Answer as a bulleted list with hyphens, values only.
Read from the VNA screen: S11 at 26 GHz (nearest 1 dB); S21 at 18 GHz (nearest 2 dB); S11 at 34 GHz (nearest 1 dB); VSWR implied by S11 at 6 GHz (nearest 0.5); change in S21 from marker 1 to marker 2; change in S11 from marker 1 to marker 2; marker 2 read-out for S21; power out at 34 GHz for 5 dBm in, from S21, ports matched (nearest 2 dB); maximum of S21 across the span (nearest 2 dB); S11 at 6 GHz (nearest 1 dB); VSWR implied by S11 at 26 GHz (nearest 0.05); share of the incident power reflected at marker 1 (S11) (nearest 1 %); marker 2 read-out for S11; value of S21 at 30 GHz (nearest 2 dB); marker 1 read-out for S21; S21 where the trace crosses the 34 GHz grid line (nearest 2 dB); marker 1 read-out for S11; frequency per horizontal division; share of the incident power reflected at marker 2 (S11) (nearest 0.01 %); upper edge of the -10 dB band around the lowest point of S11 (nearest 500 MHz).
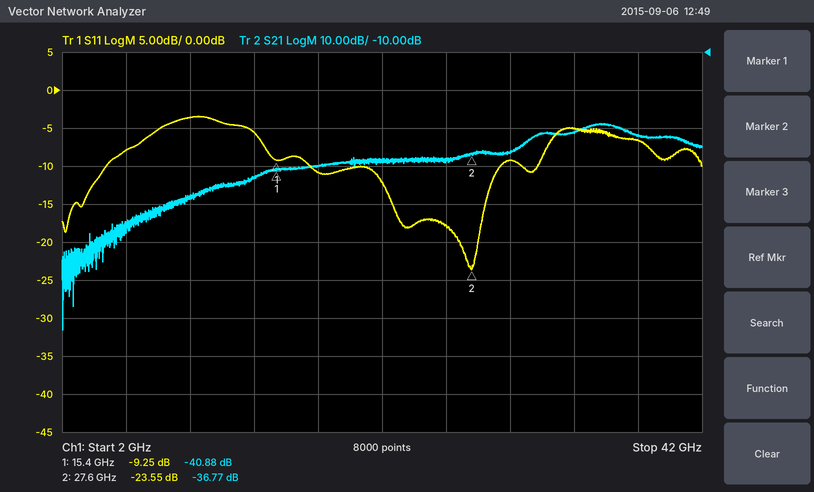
- -18 dB
- -40 dB
- -5 dB
- 2.5
- 4.11 dB
- -14.30 dB
- -36.77 dB
- -26 dBm
- -28 dB
- -8 dB
- 1.30
- 12 %
- -23.55 dB
- -36 dB
- -40.88 dB
- -32 dB
- -9.25 dB
- 4 GHz
- 0.44 %
- 29.5 GHz
